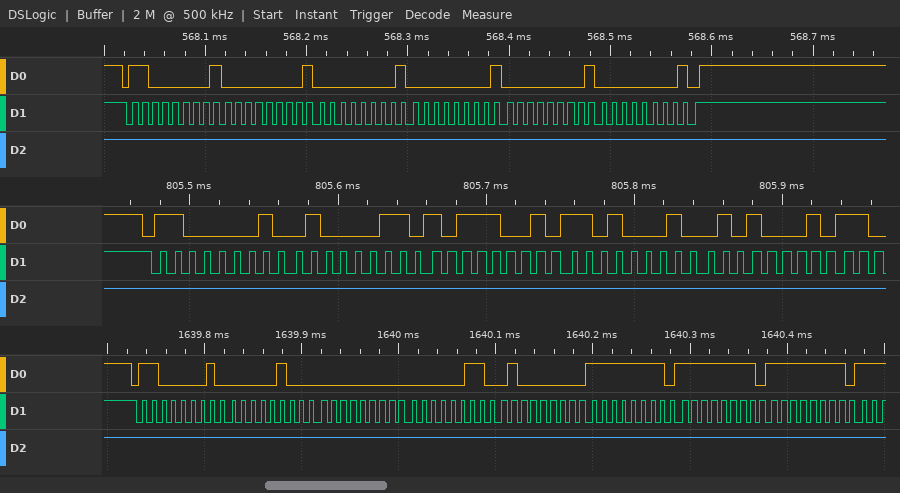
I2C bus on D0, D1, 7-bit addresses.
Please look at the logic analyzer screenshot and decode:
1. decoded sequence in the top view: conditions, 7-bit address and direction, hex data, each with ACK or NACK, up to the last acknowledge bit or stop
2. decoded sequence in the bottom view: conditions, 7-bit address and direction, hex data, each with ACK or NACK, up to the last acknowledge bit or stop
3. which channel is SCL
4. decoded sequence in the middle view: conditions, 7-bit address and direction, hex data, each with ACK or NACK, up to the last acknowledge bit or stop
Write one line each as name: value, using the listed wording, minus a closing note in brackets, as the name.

decoded sequence in the top view: conditions, 7-bit address and direction, hex data, each with ACK or NACK, up to the last acknowledge bit or stop: start, address 60 write NACK, 00 NACK, 00 NACK, 00 NACK, 00 NACK, 00 NACK, stop
decoded sequence in the bottom view: conditions, 7-bit address and direction, hex data, each with ACK or NACK, up to the last acknowledge bit or stop: start, address 60 read ACK, 04 ACK, 00 ACK, 03 ACK, 40 ACK, FF ACK, FF ACK, FF ACK
which channel is SCL: D1
decoded sequence in the middle view: conditions, 7-bit address and direction, hex data, each with ACK or NACK, up to the last acknowledge bit or stop: start, address 60 read ACK, 43 ACK, B9 ACK, D1 ACK, 51 ACK
